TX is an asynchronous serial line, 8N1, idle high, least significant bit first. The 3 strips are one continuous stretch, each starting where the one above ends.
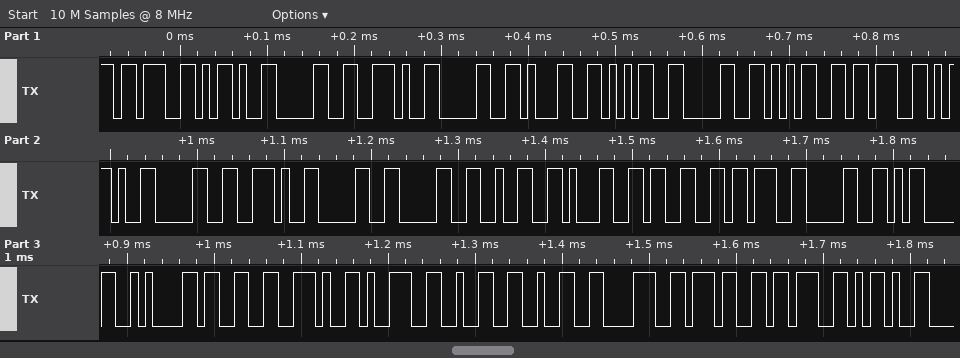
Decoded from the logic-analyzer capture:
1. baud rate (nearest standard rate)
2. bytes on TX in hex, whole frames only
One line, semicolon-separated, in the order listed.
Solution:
115200 baud; 3B 2D 30 2E 30 31 35 30 35 3B 2D 30 2E 30 30 32 31 33 3B 30 0D 0A 33 2E 39 32 32 38 37 3B 2D
